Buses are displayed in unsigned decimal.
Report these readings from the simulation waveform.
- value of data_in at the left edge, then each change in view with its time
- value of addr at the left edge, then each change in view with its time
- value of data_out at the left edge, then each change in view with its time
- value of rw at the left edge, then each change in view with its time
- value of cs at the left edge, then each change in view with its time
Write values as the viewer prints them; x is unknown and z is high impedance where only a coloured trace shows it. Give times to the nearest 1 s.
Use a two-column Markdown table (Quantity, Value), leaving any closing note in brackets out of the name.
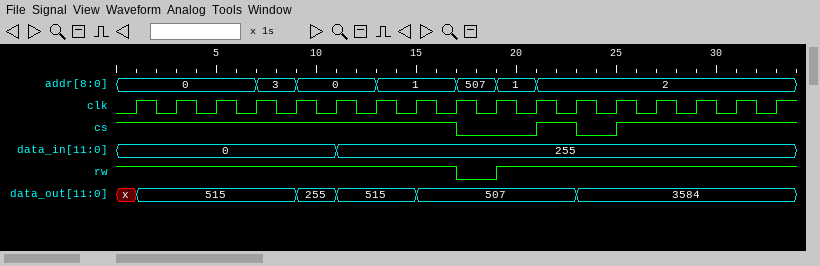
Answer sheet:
| Quantity | Value |
|---|---|
| value of data_in at the left edge, then each change in view with its time | 0, 255 at 11 s |
| value of addr at the left edge, then each change in view with its time | 0, 3 at 7 s, 0 at 9 s, 1 at 13 s, 507 at 17 s, 1 at 19 s, 2 at 21 s |
| value of data_out at the left edge, then each change in view with its time | x, 515 at 1 s, 255 at 9 s, 515 at 11 s, 507 at 15 s, 3584 at 23 s |
| value of rw at the left edge, then each change in view with its time | 1, 0 at 17 s, 1 at 19 s |
| value of cs at the left edge, then each change in view with its time | 1, 0 at 17 s, 1 at 21 s, 0 at 23 s, 1 at 25 s |
